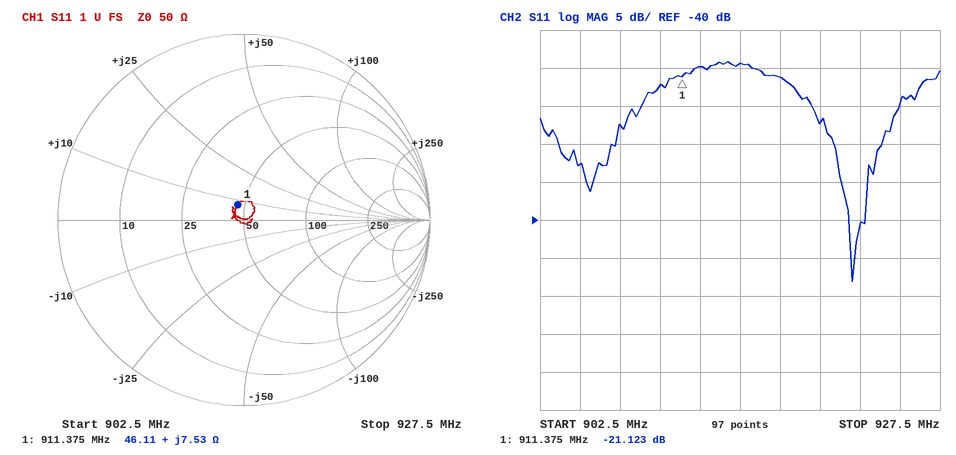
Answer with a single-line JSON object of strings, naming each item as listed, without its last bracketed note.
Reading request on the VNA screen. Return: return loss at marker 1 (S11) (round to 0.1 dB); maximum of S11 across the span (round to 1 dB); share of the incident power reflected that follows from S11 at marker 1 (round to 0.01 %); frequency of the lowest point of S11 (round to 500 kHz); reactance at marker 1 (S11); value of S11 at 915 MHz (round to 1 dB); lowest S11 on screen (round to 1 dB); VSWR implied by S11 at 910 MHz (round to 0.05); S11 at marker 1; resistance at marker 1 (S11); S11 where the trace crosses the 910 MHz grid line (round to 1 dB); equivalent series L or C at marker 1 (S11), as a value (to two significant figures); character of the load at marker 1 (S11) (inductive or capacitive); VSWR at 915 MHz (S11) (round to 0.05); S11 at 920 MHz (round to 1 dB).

{"return loss at marker 1 (S11)": "21.1 dB", "maximum of S11 across the span": "-19 dB", "share of the incident power reflected that follows from S11 at marker 1": "0.77 %", "frequency of the lowest point of S11": "922.0 MHz", "reactance at marker 1": "+7.53 Ω", "value of S11 at 915 MHz": "-19 dB", "lowest S11 on screen": "-48 dB", "VSWR implied by S11 at 910 MHz": "1.15", "S11 at marker 1": "-21.123 dB", "resistance at marker 1": "46.11 Ω", "S11 where the trace crosses the 910 MHz grid line": "-22 dB", "equivalent series L or C at marker 1 (S11), as a value": "1.3 nH", "character of the load at marker 1 (S11)": "inductive", "VSWR at 915 MHz (S11)": "1.25", "S11 at 920 MHz": "-27 dB"}
